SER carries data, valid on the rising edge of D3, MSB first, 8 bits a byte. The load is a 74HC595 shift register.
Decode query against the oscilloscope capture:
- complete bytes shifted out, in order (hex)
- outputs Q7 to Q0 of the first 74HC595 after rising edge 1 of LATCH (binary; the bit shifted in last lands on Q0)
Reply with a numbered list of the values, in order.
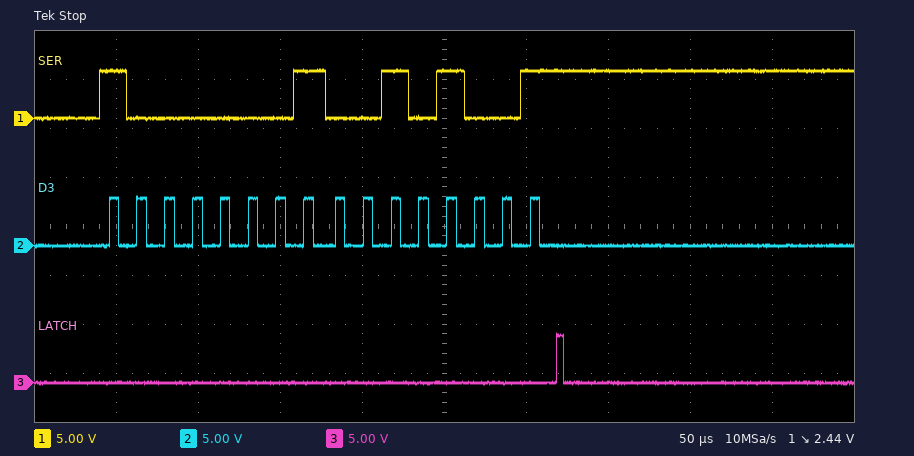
1. 81 29
2. 00101001
